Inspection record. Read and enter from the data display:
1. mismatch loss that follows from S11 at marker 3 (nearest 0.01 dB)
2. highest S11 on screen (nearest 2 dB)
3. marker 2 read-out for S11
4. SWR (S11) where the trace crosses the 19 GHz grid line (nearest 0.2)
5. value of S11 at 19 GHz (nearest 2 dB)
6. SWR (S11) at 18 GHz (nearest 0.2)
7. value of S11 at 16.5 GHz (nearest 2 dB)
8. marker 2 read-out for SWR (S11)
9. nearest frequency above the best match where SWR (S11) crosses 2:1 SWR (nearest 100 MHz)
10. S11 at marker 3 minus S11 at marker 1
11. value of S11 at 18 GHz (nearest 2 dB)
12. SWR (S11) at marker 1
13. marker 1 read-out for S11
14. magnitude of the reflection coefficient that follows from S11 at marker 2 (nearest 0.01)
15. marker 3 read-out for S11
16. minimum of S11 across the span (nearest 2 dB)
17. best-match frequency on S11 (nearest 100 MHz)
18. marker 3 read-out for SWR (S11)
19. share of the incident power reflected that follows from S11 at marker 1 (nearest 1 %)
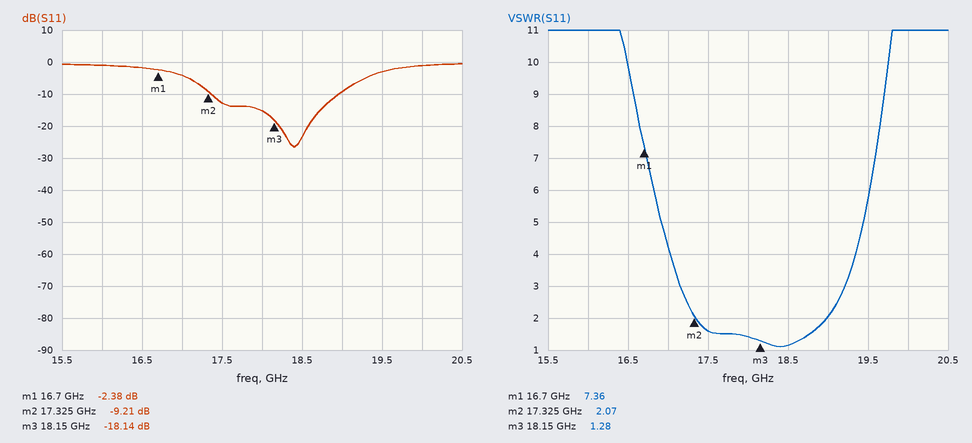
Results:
0.07 dB
0 dB
-9.21 dB
2.0
-10 dB
1.4
-2 dB
2.07
19.0 GHz
-15.76 dB
-16 dB
7.36
-2.38 dB
0.35
-18.14 dB
-26 dB
18.4 GHz
1.28
58 %
